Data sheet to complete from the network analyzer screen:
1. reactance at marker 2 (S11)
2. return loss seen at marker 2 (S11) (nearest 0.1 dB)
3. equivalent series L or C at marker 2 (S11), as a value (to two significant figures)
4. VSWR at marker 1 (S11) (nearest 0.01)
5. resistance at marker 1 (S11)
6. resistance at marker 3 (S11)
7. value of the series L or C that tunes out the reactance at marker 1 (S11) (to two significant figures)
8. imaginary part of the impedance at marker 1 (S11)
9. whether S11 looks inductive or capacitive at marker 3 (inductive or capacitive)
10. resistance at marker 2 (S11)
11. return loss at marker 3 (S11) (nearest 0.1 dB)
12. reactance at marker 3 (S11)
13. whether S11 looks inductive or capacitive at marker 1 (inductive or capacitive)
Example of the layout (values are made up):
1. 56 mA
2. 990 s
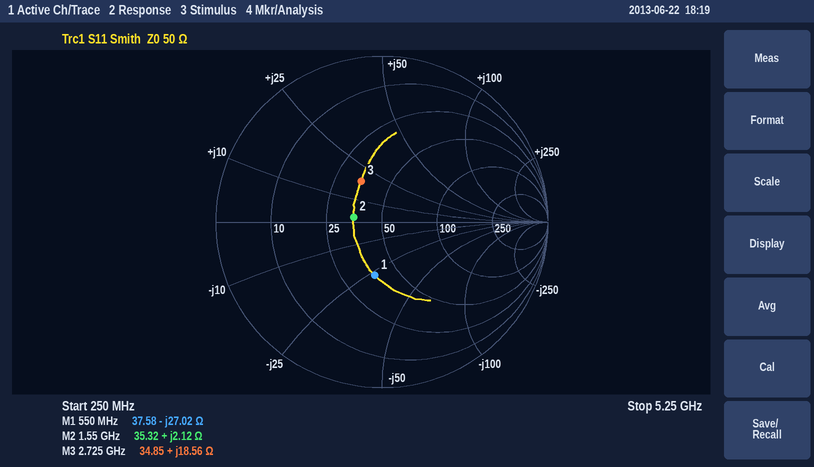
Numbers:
1. +2.12 Ω
2. 15.2 dB
3. 220 pH
4. 1.96
5. 37.58 Ω
6. 34.85 Ω
7. 7.8 nH
8. -27.02 Ω
9. inductive
10. 35.32 Ω
11. 11.2 dB
12. +18.56 Ω
13. capacitive
